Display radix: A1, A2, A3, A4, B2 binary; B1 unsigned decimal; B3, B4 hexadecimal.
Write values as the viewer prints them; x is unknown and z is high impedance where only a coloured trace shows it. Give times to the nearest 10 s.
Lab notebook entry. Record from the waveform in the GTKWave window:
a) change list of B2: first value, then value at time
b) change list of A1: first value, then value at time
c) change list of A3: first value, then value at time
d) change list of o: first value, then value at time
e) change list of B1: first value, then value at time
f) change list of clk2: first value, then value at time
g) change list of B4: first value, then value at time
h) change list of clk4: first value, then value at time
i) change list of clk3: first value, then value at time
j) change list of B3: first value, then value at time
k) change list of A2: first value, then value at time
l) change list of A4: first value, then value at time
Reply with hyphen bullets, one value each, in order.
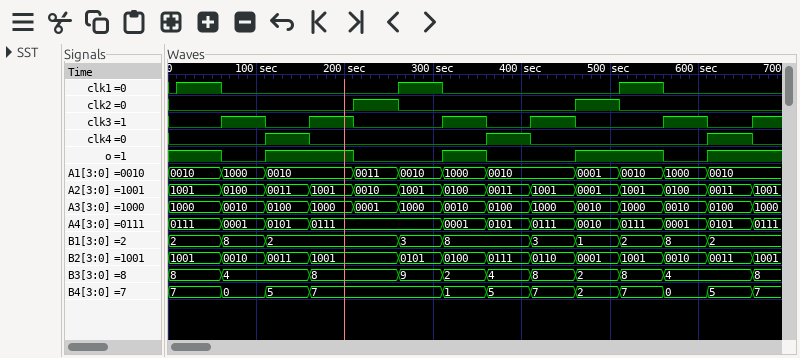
- 1001, 0010 at 60 s, 0011 at 110 s, 1001 at 160 s, 0101 at 260 s, 0100 at 310 s, 0111 at 360 s, 0110 at 410 s, 0001 at 460 s, 1001 at 510 s, 0010 at 560 s, 0011 at 610 s, 1001 at 660 s
- 0010, 1000 at 60 s, 0010 at 110 s, 0011 at 210 s, 0010 at 260 s, 1000 at 310 s, 0010 at 360 s, 0001 at 460 s, 0010 at 510 s, 1000 at 560 s, 0010 at 610 s
- 1000, 0010 at 60 s, 0100 at 110 s, 1000 at 160 s, 0001 at 210 s, 1000 at 260 s, 0010 at 310 s, 0100 at 360 s, 1000 at 410 s, 0010 at 460 s, 1000 at 510 s, 0010 at 560 s, 0100 at 610 s, 1000 at 660 s
- 1, 0 at 60 s, 1 at 110 s, 0 at 210 s, 1 at 310 s, 0 at 360 s, 1 at 460 s, 0 at 560 s, 1 at 610 s
- 2, 8 at 60 s, 2 at 110 s, 3 at 260 s, 8 at 310 s, 3 at 410 s, 1 at 460 s, 2 at 510 s, 8 at 560 s, 2 at 610 s
- 0, 1 at 210 s, 0 at 260 s, 1 at 460 s, 0 at 510 s
- 7, 0 at 60 s, 5 at 110 s, 7 at 160 s, 1 at 310 s, 5 at 360 s, 7 at 410 s, 2 at 460 s, 7 at 510 s, 0 at 560 s, 5 at 610 s, 7 at 660 s
- 0, 1 at 110 s, 0 at 160 s, 1 at 360 s, 0 at 410 s, 1 at 610 s, 0 at 660 s
- 0, 1 at 60 s, 0 at 110 s, 1 at 160 s, 0 at 210 s, 1 at 310 s, 0 at 360 s, 1 at 410 s, 0 at 460 s, 1 at 560 s, 0 at 610 s, 1 at 660 s
- 8, 4 at 60 s, 8 at 160 s, 9 at 260 s, 2 at 310 s, 4 at 360 s, 8 at 410 s, 2 at 460 s, 8 at 510 s, 4 at 560 s, 8 at 660 s
- 1001, 0100 at 60 s, 0011 at 110 s, 1001 at 160 s, 0010 at 210 s, 1001 at 260 s, 0100 at 310 s, 0011 at 360 s, 1001 at 410 s, 0001 at 460 s, 1001 at 510 s, 0100 at 560 s, 0011 at 610 s, 1001 at 660 s
- 0111, 0001 at 60 s, 0101 at 110 s, 0111 at 160 s, 0001 at 310 s, 0101 at 360 s, 0111 at 410 s, 0010 at 460 s, 0111 at 510 s, 0001 at 560 s, 0101 at 610 s, 0111 at 660 s
